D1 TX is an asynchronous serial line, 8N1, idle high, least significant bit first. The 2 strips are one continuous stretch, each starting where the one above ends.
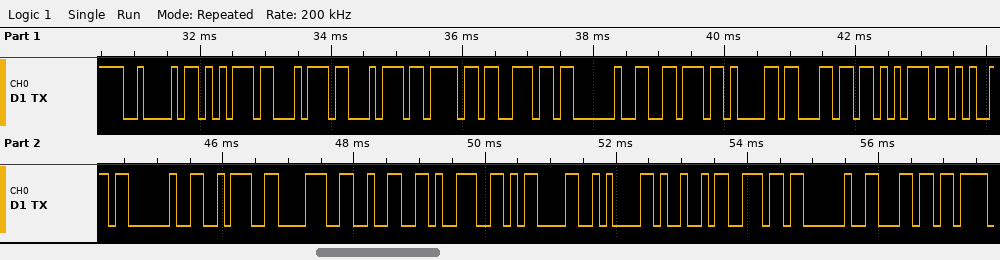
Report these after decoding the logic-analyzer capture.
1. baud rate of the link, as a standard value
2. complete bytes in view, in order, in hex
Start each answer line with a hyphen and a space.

- 9600 baud
- 42 75 74 74 6F 6E 20 76 61 6C 75 65 20 3A 38 32 39 0D 0A 49 6E 20 6C
